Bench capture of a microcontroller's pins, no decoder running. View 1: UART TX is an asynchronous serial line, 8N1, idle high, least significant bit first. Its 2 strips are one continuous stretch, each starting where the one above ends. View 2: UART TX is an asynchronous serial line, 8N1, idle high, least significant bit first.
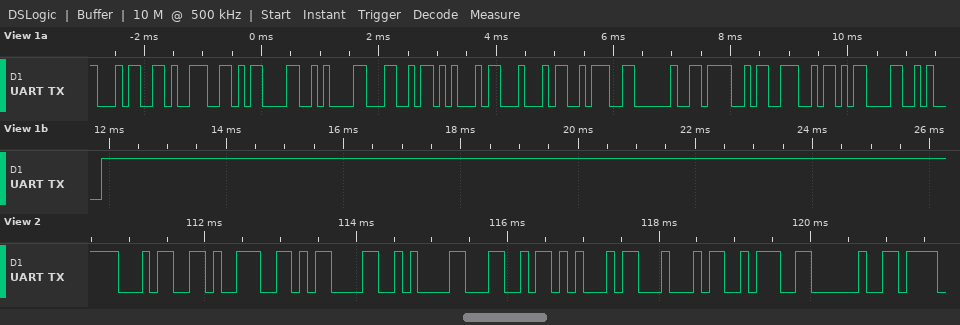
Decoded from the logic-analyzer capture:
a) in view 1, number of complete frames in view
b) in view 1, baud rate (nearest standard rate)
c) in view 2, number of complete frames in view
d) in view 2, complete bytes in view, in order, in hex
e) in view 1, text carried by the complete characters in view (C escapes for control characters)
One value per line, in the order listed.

13
9600 baud
9
34 39 0D 0A 4C 45 44 3A 20
"49\r\nLED: ON\r\n"
